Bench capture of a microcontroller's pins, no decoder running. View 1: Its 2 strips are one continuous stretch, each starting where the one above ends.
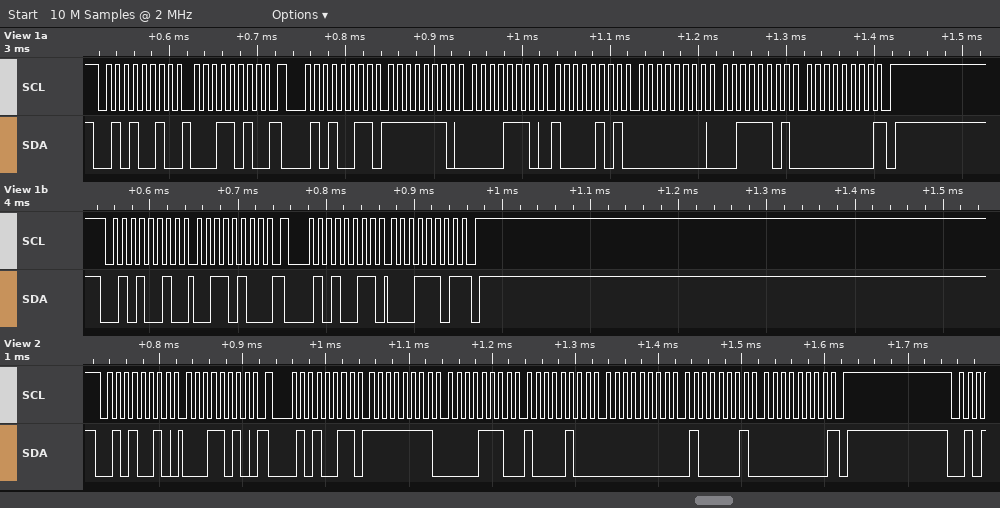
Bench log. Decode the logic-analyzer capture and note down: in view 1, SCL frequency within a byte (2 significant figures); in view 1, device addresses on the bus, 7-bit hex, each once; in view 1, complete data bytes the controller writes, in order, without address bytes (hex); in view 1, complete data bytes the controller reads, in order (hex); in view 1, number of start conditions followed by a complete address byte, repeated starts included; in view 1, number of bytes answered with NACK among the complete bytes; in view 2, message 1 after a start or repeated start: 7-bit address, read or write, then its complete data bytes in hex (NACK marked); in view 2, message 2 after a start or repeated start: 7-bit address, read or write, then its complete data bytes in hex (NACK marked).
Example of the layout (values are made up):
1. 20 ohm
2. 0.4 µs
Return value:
1. 100 kHz
2. 0x29
3. 1A 34
4. FE 0E 85 00 3D 00 1D
5. 4
6. 2
7. 0x29 write: 1A
8. 0x29 read: FF 0E 84 00 41 00 NACK
